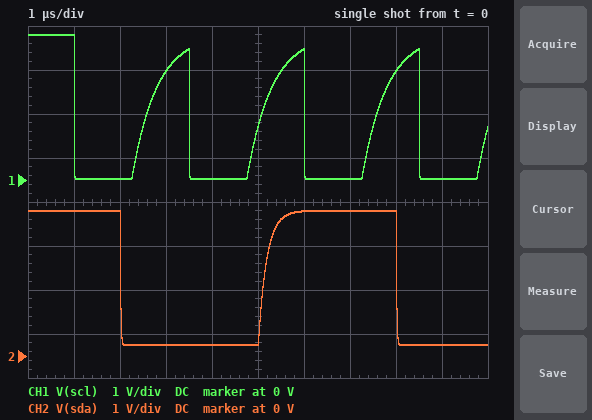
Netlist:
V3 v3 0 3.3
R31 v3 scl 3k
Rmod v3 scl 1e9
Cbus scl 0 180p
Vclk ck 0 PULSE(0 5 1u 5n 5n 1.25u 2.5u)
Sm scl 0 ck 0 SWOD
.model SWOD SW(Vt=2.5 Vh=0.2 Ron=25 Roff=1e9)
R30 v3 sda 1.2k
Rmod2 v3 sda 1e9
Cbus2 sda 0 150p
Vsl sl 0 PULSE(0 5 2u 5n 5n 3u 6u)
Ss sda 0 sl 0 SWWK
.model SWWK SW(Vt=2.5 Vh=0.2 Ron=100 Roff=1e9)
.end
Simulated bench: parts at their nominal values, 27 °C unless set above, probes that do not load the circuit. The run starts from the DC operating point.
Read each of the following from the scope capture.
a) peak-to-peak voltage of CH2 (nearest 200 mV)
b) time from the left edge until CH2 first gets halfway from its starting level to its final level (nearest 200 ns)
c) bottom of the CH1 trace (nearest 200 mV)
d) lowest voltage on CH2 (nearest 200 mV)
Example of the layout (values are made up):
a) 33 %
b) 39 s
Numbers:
a) 3.0 V
b) 2.0 µs
c) 0 V
d) 200 mV
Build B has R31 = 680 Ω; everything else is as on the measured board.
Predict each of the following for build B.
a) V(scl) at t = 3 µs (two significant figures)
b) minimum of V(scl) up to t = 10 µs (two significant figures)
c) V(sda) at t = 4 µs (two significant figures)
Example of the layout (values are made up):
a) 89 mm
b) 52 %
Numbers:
a) 3.3 V
b) 120 mV
c) 250 mV
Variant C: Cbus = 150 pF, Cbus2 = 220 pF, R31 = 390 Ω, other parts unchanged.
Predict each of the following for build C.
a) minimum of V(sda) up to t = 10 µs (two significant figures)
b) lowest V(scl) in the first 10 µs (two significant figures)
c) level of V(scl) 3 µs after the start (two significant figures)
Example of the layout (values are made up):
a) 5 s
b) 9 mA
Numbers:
a) 250 mV
b) 200 mV
c) 3.3 V
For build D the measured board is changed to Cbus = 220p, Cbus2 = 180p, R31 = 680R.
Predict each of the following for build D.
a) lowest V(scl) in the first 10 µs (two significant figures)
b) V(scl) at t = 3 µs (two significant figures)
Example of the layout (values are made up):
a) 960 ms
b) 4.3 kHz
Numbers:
a) 120 mV
b) 3.3 V
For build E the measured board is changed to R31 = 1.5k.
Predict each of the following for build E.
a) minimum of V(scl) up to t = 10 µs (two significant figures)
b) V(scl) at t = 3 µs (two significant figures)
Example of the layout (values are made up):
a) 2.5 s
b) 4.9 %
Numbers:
a) 54 mV
b) 3.1 V
